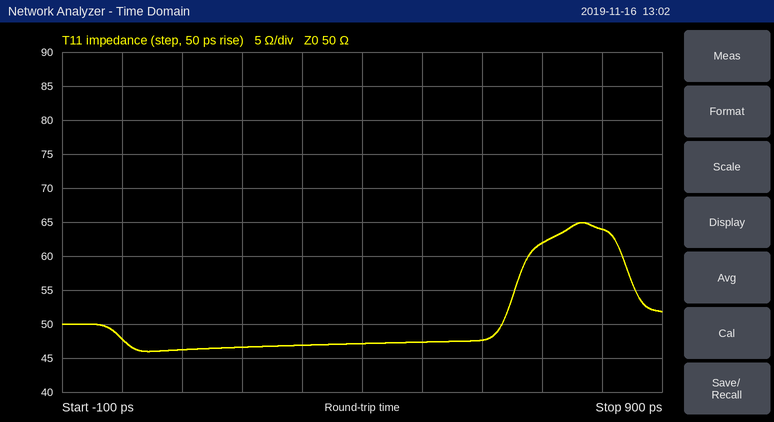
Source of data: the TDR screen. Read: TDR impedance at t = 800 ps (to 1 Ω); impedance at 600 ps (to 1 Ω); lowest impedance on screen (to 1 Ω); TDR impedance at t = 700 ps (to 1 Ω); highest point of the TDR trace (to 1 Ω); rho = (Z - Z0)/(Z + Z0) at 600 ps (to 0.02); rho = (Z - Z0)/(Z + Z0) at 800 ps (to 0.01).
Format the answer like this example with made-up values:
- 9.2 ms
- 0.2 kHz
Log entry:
- 64 Ω
- 48 Ω
- 46 Ω
- 62 Ω
- 65 Ω
- -0.02
- +0.12
